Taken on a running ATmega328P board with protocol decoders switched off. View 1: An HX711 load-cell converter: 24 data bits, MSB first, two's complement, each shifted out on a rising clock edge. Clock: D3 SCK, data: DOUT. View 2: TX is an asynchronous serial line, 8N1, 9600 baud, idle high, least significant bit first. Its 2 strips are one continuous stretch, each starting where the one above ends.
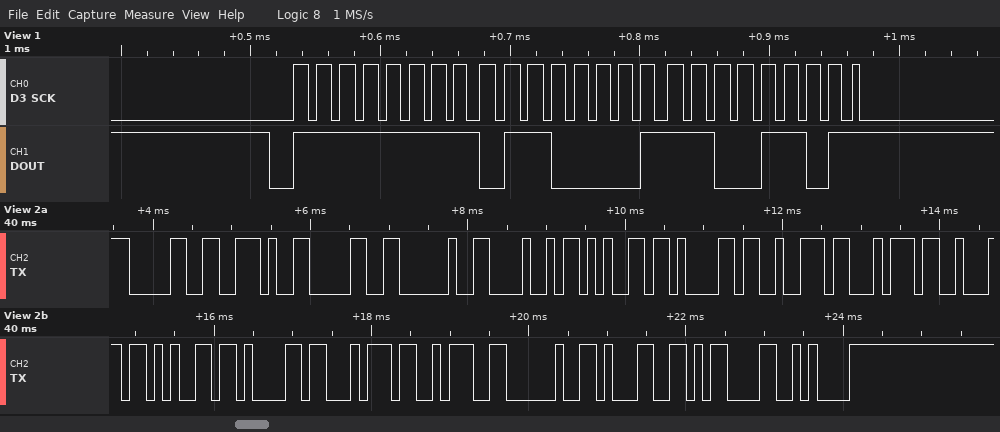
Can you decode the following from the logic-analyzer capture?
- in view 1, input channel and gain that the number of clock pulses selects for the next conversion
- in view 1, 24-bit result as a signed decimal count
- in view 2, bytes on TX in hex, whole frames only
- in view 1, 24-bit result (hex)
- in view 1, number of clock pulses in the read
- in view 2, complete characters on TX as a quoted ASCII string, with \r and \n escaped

channel A, gain 128
-40499
30 2E 30 20 48 65 61 72 74 62 65 61 74 3A 20 31 0D 0A
0xFF61CD
25
"0.0 Heartbeat: 1\r\n"
